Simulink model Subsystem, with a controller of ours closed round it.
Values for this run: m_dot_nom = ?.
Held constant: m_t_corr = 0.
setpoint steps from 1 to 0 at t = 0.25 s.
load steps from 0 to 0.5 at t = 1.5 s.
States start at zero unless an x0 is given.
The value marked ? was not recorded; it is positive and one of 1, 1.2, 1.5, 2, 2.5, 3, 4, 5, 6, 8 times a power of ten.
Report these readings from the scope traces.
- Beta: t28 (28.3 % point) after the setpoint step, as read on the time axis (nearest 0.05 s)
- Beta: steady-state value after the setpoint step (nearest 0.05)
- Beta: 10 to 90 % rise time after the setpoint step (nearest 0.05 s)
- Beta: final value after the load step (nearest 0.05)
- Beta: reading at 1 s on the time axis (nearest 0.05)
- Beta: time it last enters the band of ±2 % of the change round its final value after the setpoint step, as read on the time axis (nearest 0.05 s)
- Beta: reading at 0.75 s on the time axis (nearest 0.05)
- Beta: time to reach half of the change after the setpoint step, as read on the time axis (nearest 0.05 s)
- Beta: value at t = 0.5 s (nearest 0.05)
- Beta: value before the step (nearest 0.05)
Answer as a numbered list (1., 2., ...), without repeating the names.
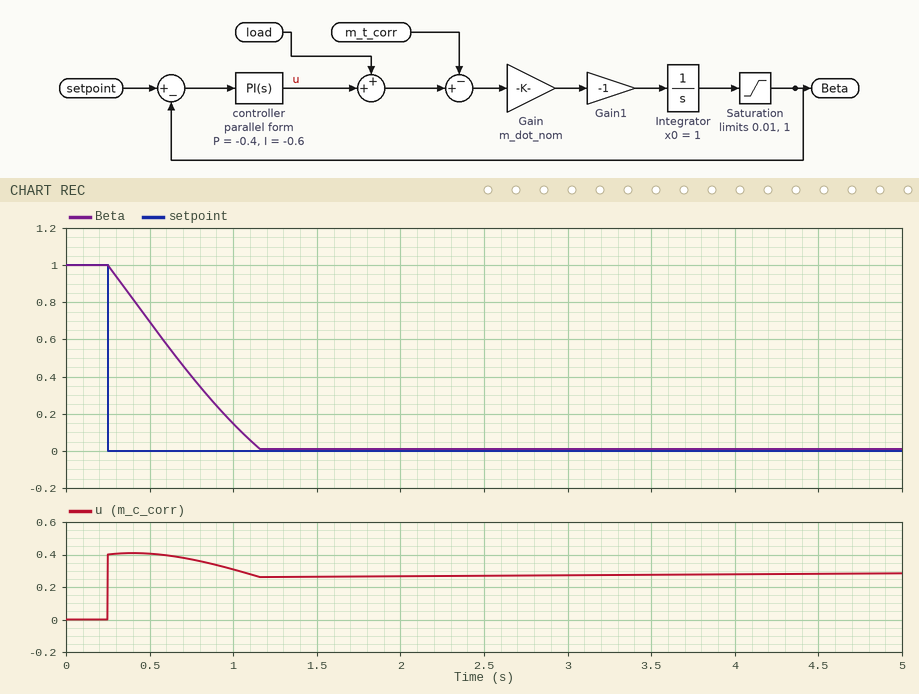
1. 0.50 s
2. 0.00
3. 0.70 s
4. 0.00
5. 0.15
6. 1.15 s
7. 0.40
8. 0.65 s
9. 0.70
10. 1.00
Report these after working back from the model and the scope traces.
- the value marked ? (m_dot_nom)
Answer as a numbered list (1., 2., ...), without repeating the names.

1. 3
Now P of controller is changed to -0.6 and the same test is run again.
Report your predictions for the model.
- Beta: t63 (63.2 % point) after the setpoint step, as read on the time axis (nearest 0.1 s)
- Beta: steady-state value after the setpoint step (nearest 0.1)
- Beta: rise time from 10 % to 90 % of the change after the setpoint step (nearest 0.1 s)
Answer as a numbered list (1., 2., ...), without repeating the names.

1. 0.7 s
2. 0.0
3. 0.6 s
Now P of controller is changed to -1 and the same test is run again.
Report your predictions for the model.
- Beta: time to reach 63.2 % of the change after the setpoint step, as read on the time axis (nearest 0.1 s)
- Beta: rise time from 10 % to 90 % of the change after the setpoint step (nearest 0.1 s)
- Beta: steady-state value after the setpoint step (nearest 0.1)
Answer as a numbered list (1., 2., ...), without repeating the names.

1. 0.5 s
2. 0.5 s
3. 0.0
